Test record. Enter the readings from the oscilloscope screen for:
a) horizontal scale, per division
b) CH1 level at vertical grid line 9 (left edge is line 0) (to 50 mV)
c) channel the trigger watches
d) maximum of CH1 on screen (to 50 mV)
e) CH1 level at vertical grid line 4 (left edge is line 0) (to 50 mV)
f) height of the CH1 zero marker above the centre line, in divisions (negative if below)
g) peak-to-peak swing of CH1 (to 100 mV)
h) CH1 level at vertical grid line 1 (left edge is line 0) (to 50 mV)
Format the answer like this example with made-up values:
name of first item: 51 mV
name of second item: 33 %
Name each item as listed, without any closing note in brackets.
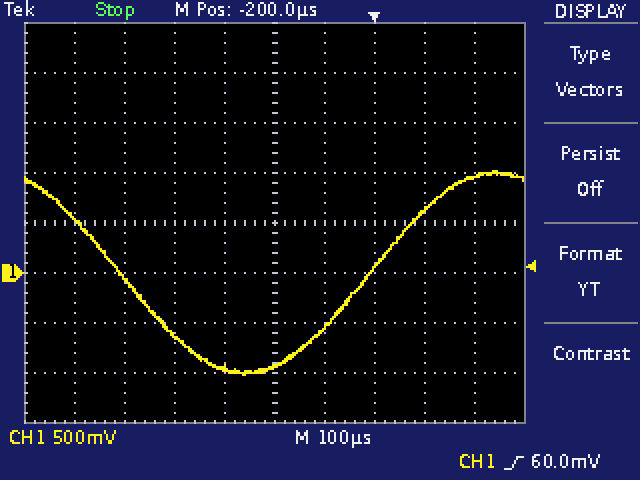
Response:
horizontal scale, per division: 100 µs
CH1 level at vertical grid line 9 (left edge is line 0): 950 mV
channel the trigger watches: CH1
maximum of CH1 on screen: 1.00 V
CH1 level at vertical grid line 4 (left edge is line 0): -950 mV
height of the CH1 zero marker above the centre line, in divisions: -1.0 div
peak-to-peak swing of CH1: 2.00 V
CH1 level at vertical grid line 1 (left edge is line 0): 550 mV
